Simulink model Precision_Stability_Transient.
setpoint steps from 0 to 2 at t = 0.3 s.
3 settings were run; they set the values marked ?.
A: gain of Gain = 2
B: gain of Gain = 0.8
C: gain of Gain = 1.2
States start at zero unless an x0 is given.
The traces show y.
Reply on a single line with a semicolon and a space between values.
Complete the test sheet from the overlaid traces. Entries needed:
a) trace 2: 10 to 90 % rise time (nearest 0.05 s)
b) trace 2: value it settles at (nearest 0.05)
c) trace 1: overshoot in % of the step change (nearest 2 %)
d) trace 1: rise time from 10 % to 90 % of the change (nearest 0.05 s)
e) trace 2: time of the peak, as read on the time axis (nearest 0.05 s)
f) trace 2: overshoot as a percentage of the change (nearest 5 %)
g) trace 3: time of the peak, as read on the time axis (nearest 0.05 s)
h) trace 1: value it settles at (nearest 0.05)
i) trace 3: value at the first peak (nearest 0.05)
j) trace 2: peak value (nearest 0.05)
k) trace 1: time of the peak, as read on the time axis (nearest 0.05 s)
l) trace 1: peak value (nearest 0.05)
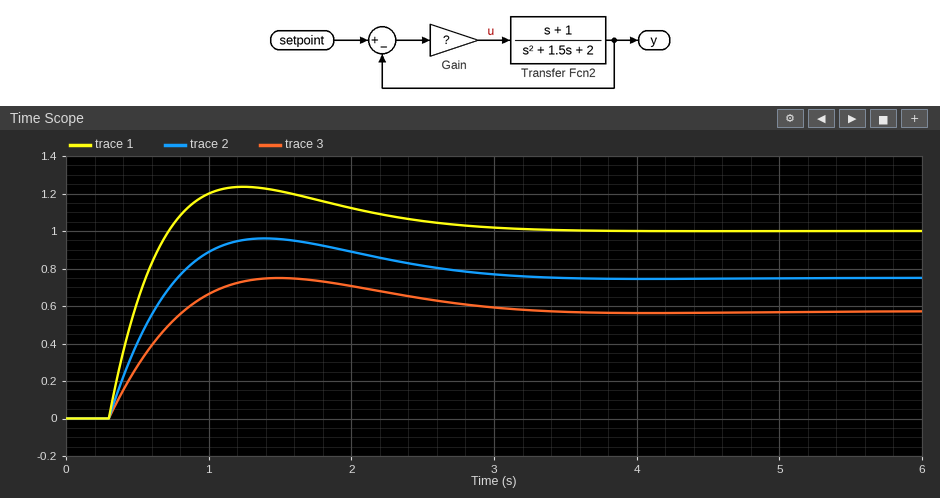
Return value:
0.35 s; 0.75; 24 %; 0.30 s; 1.40 s; 30 %; 1.50 s; 1.00; 0.75; 0.95; 1.25 s; 1.25
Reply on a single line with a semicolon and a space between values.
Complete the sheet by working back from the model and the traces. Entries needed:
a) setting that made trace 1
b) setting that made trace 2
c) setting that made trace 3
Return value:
A; C; B
